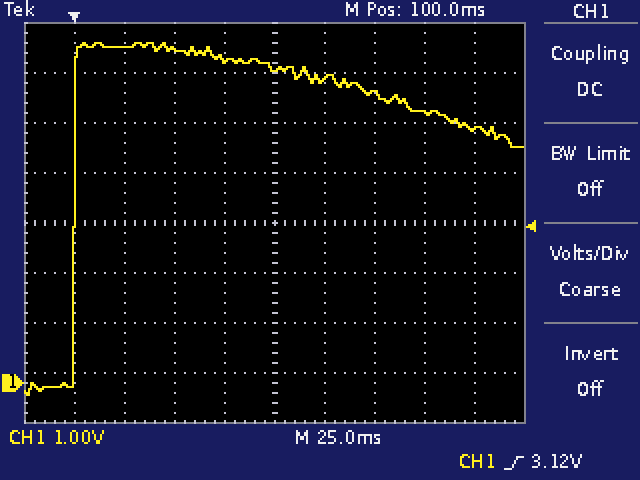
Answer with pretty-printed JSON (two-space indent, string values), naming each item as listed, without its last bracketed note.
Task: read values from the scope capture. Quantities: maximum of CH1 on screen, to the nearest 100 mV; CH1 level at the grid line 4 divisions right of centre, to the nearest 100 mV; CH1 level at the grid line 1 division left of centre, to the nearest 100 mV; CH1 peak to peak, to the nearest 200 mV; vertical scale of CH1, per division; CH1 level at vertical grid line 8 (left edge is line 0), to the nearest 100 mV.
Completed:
{
  "maximum of CH1 on screen, to the nearest 100 mV": "6.8 V",
  "CH1 level at the grid line 4 divisions right of centre, to the nearest 100 mV": "5.1 V",
  "CH1 level at the grid line 1 division left of centre, to the nearest 100 mV": "6.5 V",
  "CH1 peak to peak, to the nearest 200 mV": "7.0 V",
  "vertical scale of CH1, per division": "1 V",
  "CH1 level at vertical grid line 8 (left edge is line 0), to the nearest 100 mV": "5.4 V"
}
